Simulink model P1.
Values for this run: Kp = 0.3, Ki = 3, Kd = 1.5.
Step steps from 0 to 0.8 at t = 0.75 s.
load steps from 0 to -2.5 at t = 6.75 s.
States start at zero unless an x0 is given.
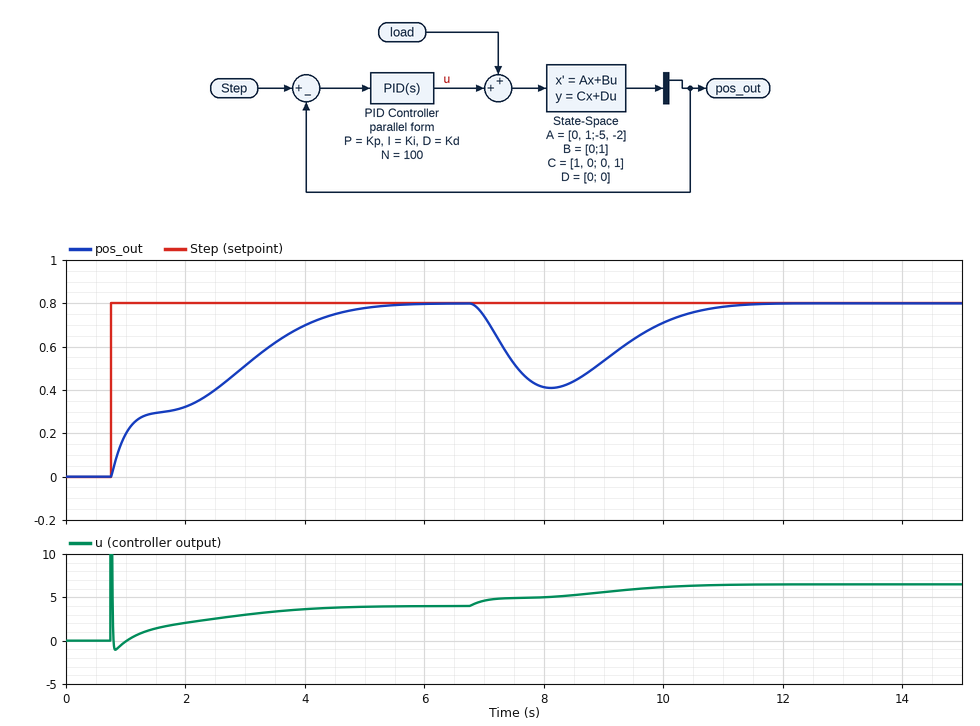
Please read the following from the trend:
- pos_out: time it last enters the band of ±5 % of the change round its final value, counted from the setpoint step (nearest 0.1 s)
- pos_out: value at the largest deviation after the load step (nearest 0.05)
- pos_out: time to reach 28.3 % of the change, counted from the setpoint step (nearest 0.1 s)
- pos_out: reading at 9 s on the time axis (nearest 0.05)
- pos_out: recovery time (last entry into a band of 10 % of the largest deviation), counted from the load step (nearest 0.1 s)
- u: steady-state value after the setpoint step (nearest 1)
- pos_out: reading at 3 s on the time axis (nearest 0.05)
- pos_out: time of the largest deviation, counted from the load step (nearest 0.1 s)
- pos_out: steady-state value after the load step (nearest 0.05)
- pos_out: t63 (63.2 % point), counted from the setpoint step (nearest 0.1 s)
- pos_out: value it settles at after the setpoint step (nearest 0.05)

3.9 s
0.40
0.3 s
0.55
3.8 s
4
0.50
1.4 s
0.80
2.2 s
0.80
